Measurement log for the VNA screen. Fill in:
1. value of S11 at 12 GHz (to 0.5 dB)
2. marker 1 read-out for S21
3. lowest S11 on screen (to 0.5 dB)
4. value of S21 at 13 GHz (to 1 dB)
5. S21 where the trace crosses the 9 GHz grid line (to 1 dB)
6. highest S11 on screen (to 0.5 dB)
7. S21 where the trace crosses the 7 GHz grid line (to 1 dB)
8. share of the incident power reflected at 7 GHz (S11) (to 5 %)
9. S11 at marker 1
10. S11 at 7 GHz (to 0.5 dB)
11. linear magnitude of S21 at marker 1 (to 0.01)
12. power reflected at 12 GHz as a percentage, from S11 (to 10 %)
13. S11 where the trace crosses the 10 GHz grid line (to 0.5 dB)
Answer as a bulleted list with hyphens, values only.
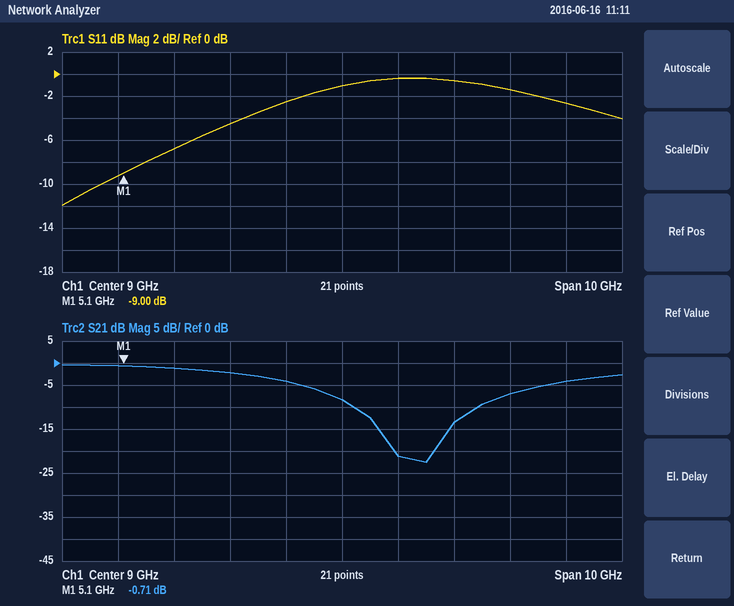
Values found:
- -1.5 dB
- -0.71 dB
- -12.0 dB
- -4 dB
- -8 dB
- -0.5 dB
- -2 dB
- 35 %
- -9.00 dB
- -4.5 dB
- 0.92
- 70 %
- -0.5 dB
